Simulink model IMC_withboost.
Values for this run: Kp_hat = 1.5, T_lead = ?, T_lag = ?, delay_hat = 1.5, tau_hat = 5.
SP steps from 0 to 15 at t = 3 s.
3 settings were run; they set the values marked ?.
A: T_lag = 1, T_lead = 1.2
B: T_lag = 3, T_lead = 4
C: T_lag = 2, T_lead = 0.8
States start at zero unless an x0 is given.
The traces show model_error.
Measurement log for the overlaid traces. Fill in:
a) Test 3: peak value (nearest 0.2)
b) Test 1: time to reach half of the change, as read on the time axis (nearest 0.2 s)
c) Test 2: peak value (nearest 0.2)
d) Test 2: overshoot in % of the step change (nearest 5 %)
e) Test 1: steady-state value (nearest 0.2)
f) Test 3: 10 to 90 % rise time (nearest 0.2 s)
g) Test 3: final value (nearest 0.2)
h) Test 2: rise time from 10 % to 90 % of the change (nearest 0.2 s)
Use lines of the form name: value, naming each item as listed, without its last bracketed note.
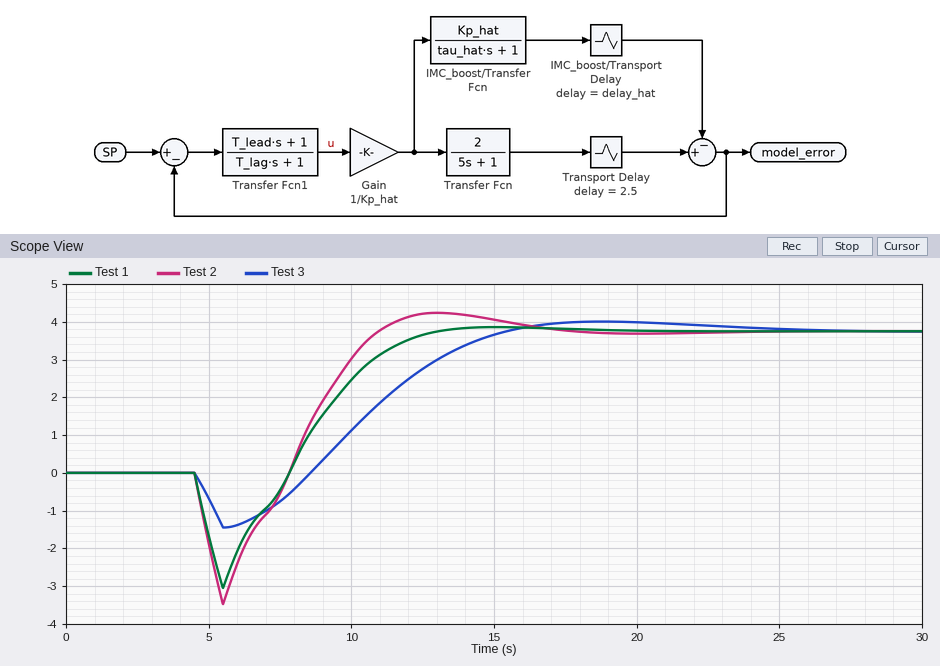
Test 3: peak value: 4.0
Test 1: time to reach half of the change, as read on the time axis: 9.4 s
Test 2: peak value: 4.2
Test 2: overshoot in % of the step change: 15 %
Test 1: steady-state value: 3.8
Test 3: 10 to 90 % rise time: 5.0 s
Test 3: final value: 3.8
Test 2: rise time from 10 % to 90 % of the change: 2.4 s
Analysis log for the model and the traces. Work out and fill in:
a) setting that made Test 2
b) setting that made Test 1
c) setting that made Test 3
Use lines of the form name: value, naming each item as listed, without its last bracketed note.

setting that made Test 2: B
setting that made Test 1: A
setting that made Test 3: C
